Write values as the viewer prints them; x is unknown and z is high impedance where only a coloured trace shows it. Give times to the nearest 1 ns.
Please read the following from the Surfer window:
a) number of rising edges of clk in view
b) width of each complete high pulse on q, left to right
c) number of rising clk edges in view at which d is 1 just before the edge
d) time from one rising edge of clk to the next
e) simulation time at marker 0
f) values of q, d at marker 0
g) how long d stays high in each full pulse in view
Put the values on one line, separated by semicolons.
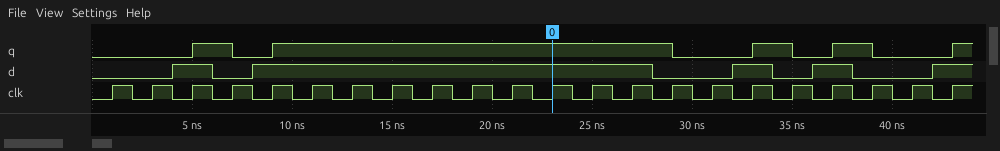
22; 2 ns, 20 ns, 2 ns, 2 ns; 14; 2 ns; 23 ns; q=1, d=1; 2 ns, 20 ns, 2 ns, 2 ns
